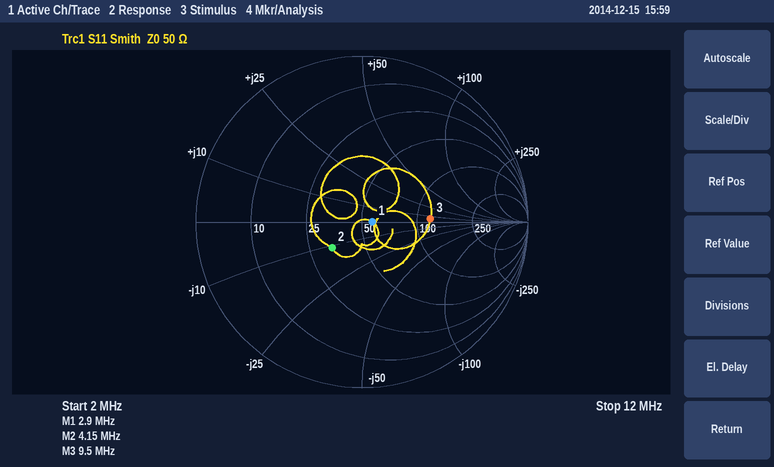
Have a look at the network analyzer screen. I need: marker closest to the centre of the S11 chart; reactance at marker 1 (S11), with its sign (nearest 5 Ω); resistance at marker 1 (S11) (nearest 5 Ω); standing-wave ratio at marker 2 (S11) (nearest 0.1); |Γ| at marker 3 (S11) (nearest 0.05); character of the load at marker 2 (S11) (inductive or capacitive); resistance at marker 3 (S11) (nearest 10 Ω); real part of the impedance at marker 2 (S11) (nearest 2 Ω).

marker 1
0 Ω
55 Ω
1.6
0.40
capacitive
120 Ω
34 Ω
